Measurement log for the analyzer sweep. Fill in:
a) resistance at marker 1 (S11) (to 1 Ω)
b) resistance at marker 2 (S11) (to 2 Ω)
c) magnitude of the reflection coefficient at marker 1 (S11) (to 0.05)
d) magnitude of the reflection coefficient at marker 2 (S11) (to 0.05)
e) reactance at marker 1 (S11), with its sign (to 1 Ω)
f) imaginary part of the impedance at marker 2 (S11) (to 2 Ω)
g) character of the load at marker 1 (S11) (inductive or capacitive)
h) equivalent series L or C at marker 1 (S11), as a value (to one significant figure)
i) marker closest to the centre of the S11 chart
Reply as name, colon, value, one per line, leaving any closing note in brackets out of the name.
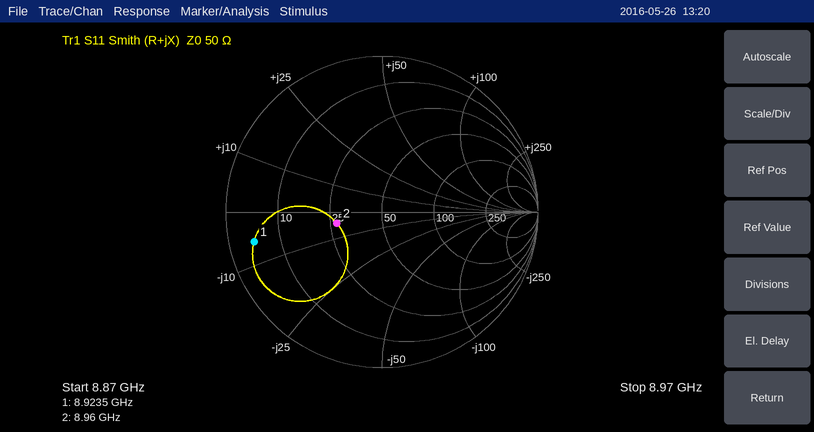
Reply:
resistance at marker 1 (S11): 4 Ω
resistance at marker 2 (S11): 28 Ω
magnitude of the reflection coefficient at marker 1 (S11): 0.85
magnitude of the reflection coefficient at marker 2 (S11): 0.30
reactance at marker 1 (S11), with its sign: -6 Ω
imaginary part of the impedance at marker 2 (S11): -4 Ω
character of the load at marker 1 (S11): capacitive
equivalent series L or C at marker 1 (S11), as a value: 3 pF
marker closest to the centre of the S11 chart: marker 2
